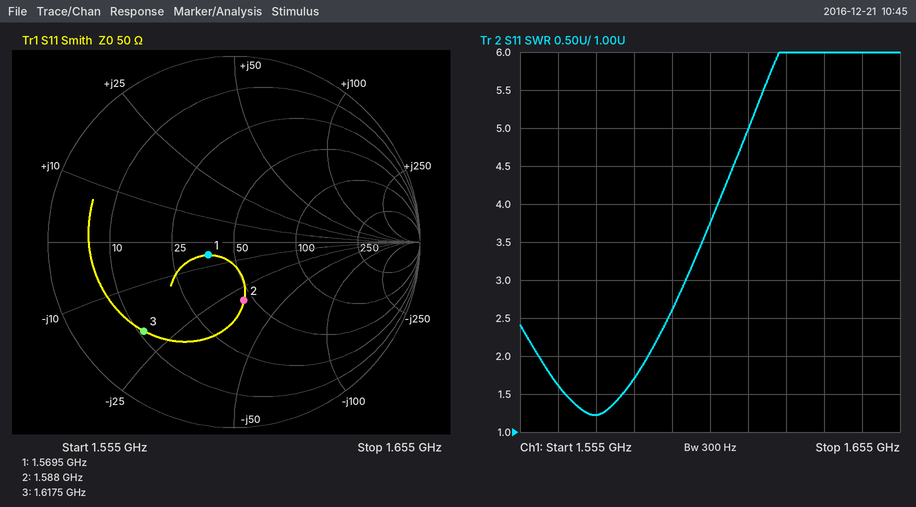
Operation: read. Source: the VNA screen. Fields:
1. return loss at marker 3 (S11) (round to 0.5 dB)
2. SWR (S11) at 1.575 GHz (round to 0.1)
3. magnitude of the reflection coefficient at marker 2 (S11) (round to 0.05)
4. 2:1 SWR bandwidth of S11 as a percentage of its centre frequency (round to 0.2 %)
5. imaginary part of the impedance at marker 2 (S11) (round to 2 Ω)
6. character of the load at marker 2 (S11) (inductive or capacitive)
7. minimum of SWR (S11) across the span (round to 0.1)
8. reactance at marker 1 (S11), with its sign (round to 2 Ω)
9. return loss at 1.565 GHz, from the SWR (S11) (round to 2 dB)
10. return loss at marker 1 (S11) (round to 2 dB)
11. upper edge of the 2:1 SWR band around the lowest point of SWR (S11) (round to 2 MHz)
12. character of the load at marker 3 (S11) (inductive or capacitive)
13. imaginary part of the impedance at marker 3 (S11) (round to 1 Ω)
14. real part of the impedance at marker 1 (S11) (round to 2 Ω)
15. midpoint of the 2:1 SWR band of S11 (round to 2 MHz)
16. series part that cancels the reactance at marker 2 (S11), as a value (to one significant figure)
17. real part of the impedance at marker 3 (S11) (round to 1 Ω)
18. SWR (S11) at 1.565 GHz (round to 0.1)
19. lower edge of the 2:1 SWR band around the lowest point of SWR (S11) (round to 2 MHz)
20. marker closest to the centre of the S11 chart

3.5 dB
1.2
0.30
1.8 %
-32 Ω
capacitive
1.2
-6 Ω
12 dB
16 dB
1.588 GHz
capacitive
-20 Ω
38 Ω
1.574 GHz
3 nH
11 Ω
1.6
1.560 GHz
marker 1
